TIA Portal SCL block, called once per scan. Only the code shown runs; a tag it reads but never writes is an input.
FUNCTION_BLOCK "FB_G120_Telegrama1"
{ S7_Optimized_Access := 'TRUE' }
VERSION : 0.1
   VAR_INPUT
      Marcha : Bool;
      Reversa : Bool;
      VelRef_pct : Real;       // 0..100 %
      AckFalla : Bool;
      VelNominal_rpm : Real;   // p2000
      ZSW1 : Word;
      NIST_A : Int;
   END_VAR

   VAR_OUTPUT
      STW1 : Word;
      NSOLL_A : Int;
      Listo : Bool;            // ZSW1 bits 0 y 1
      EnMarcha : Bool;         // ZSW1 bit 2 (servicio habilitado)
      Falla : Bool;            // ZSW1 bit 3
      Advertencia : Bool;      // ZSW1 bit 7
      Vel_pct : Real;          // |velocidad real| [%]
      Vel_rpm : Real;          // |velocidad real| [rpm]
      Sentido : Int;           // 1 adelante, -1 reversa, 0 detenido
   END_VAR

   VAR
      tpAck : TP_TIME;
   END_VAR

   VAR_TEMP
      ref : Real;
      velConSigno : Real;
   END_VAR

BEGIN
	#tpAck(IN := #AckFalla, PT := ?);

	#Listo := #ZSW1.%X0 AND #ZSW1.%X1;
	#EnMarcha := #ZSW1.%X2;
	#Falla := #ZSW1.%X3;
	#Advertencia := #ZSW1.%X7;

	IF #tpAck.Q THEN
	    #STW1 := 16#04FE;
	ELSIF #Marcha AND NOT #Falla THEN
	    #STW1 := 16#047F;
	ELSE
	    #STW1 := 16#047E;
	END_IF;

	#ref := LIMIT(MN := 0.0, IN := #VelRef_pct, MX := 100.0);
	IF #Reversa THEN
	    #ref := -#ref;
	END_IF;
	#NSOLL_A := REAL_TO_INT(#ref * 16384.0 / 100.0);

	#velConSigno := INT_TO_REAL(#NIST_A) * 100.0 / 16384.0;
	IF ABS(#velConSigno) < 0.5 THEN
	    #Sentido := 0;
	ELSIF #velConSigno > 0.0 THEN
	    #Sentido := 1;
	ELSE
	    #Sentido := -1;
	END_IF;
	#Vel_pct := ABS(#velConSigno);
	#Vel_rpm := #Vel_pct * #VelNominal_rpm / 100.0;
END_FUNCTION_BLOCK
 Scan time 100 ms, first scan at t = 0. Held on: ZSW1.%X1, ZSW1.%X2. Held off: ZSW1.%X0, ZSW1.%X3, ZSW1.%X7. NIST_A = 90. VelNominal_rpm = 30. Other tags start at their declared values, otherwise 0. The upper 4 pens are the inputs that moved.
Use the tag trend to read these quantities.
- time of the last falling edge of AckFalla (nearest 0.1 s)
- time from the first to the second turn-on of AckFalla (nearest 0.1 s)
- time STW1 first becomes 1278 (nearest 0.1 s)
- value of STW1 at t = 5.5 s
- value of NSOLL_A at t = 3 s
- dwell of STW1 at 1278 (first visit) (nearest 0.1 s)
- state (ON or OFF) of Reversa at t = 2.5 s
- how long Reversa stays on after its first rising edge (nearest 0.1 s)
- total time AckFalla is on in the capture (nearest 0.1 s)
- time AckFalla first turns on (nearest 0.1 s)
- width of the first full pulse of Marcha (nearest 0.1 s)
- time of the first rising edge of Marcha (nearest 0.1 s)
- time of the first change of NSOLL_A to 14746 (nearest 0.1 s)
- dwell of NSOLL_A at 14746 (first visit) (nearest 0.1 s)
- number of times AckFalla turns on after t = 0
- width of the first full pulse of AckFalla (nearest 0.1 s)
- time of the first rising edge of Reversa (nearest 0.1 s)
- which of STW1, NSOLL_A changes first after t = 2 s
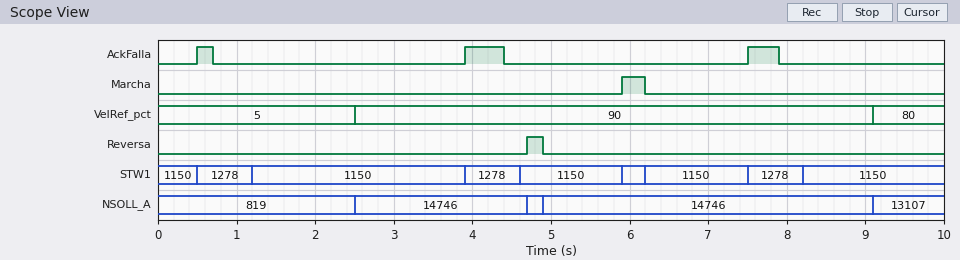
7.9 s
3.4 s
0.5 s
1150
14746
0.7 s
OFF
0.2 s
1.1 s
0.5 s
0.3 s
5.9 s
2.5 s
2.2 s
3
0.2 s
4.7 s
NSOLL_A
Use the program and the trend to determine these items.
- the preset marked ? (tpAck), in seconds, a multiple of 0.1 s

0.7 s
